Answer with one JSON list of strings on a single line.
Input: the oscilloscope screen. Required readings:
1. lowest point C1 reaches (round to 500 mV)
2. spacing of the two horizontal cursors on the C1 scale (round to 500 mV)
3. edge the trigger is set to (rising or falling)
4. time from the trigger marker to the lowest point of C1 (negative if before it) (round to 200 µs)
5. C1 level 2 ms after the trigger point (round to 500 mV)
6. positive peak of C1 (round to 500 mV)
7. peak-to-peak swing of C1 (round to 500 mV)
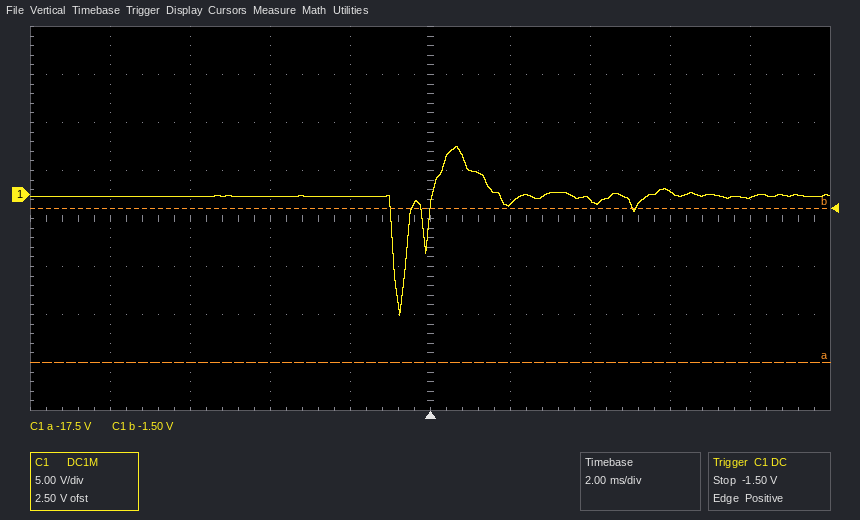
["-12.5 V", "16.0 V", "rising", "-800 µs", "-1.0 V", "5.0 V", "17.5 V"]
